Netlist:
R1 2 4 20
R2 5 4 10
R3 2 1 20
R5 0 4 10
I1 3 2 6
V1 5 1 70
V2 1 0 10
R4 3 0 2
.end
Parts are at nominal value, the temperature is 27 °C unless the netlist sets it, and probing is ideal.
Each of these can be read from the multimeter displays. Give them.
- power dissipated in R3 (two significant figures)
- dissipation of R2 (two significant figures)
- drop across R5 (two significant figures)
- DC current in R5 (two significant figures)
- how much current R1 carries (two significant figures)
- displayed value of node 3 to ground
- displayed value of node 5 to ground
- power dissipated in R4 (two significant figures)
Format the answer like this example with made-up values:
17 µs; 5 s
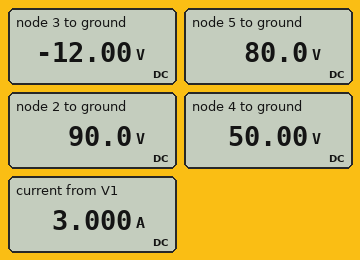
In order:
320 W; 90 W; 50 V; 5.0 A; 2.0 A; -12.00 V; 80.0 V; 72 W
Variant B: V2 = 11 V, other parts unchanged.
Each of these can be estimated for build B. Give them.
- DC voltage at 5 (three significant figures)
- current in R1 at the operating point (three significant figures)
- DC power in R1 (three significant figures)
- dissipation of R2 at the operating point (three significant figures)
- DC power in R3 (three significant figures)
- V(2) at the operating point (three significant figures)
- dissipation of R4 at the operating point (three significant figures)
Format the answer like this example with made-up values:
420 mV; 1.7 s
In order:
81.0 V; 2.01 A; 80.9 W; 92.7 W; 318 W; 90.8 V; 72.0 W
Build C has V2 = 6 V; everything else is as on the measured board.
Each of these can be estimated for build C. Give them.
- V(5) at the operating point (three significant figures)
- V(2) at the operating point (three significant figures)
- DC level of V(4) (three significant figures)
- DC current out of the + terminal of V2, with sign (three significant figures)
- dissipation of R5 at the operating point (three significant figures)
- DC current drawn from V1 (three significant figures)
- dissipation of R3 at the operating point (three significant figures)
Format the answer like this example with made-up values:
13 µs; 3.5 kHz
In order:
76.0 V; 86.9 V; 47.8 V; -1.22 A; 228 W; 2.82 A; 327 W
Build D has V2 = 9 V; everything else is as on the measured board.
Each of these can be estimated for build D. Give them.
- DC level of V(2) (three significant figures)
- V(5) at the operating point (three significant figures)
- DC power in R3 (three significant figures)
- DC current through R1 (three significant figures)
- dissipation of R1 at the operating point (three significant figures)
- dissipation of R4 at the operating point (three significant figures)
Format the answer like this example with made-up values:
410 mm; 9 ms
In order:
89.2 V; 79.0 V; 322 W; 1.99 A; 79.1 W; 72.0 W
